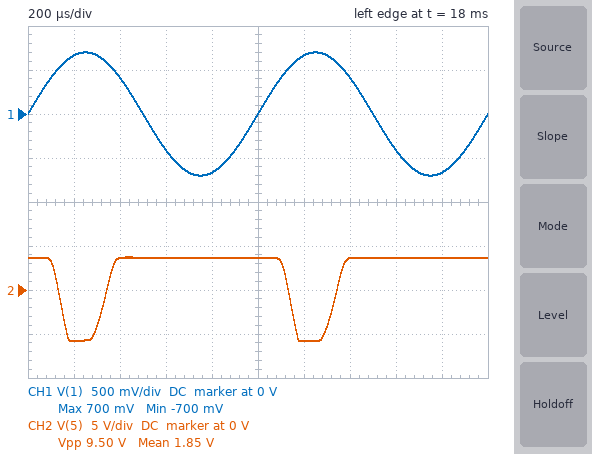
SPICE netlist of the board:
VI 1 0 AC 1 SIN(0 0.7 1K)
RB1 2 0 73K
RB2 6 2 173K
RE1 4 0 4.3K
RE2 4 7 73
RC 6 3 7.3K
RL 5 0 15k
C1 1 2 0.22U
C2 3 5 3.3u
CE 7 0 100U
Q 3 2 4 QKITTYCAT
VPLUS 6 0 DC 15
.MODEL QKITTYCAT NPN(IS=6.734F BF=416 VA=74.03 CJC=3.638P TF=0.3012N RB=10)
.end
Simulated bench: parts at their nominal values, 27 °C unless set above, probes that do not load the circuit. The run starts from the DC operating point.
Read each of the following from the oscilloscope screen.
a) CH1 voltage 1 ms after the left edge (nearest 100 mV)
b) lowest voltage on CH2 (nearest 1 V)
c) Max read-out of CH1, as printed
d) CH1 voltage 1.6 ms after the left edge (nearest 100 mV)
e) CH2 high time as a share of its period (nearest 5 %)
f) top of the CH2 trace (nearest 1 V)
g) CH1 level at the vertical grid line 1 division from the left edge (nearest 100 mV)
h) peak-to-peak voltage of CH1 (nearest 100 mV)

0 V
-6 V
700 mV
-400 mV
80 %
4 V
700 mV
1.4 V
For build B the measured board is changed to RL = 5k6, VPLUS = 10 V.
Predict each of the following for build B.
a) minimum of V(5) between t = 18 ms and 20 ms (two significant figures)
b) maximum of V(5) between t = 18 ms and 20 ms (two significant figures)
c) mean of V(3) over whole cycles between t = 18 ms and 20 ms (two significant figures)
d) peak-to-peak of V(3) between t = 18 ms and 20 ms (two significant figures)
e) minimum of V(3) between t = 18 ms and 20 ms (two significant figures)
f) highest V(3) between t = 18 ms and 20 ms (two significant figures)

-4.3 V
1.5 V
7.1 V
5.7 V
2.4 V
8.1 V
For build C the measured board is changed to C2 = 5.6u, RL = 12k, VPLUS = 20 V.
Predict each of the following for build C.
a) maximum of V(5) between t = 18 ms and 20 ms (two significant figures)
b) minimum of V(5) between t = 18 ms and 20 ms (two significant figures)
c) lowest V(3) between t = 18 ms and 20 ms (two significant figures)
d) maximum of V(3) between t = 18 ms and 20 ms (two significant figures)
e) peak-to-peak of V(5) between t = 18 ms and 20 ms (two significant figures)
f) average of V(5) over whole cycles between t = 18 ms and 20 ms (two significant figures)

5.0 V
-6.9 V
5.2 V
17 V
12 V
2.5 V
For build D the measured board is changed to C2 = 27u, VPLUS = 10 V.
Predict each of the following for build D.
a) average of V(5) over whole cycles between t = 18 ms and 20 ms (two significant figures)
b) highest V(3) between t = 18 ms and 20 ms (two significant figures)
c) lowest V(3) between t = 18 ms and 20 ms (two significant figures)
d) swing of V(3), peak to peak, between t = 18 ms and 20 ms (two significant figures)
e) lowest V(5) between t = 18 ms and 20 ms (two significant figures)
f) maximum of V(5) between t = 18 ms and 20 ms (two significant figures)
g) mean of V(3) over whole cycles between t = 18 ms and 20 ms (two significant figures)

1.4 V
8.8 V
2.3 V
6.4 V
-3.9 V
2.5 V
7.6 V
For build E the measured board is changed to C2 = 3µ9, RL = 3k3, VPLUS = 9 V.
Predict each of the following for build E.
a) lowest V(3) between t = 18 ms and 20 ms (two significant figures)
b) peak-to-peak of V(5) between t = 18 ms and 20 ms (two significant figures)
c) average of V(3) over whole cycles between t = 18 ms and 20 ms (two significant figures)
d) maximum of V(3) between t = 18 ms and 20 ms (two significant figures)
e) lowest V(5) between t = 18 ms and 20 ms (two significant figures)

2.2 V
4.7 V
5.9 V
6.8 V
-3.7 V
